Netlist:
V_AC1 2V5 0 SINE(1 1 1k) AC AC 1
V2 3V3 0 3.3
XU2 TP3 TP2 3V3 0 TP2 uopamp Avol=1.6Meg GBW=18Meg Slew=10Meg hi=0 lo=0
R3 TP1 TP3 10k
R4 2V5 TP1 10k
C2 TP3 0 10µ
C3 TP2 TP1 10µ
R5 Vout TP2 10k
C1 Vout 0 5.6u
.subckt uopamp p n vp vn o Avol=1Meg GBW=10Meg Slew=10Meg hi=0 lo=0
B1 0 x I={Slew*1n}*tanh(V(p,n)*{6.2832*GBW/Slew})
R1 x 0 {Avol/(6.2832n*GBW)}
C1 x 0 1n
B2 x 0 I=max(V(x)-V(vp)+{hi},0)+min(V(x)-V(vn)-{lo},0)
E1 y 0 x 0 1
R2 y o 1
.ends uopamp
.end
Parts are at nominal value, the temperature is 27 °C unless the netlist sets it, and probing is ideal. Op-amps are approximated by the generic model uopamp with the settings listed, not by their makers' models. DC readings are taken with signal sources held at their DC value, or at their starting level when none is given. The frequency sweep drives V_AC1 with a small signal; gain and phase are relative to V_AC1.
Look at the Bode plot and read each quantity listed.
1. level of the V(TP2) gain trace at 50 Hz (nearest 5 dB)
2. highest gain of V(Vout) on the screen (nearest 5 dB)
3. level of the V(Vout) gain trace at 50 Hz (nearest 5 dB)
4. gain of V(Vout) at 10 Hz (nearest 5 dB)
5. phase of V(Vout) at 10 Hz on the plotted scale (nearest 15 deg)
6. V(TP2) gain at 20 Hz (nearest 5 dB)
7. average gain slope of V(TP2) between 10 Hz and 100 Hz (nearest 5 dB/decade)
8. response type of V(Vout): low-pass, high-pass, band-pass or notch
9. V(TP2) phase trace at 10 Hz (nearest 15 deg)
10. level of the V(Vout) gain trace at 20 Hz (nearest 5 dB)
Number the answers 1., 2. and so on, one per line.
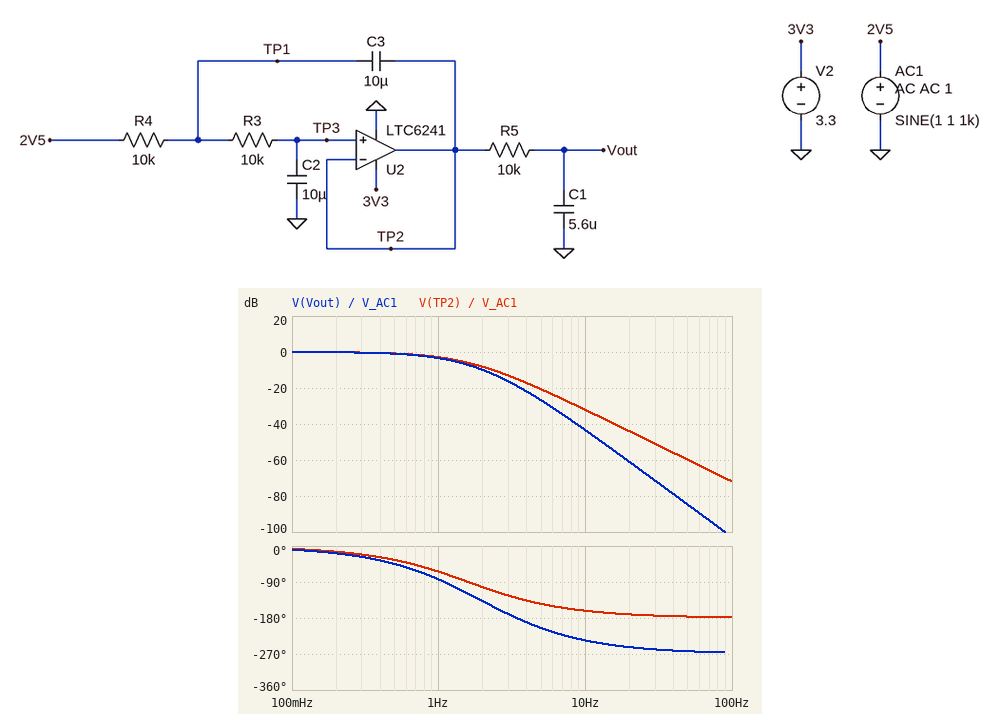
1. -60 dB
2. 0 dB
3. -85 dB
4. -45 dB
5. -240 deg
6. -45 dB
7. -40 dB/decade
8. low-pass
9. -165 deg
10. -60 dB
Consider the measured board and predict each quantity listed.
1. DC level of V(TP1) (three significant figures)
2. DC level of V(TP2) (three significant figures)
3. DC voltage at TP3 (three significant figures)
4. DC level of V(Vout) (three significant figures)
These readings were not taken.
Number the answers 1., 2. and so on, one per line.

1. 1.00 V
2. 1.00 V
3. 1.00 V
4. 1.00 V
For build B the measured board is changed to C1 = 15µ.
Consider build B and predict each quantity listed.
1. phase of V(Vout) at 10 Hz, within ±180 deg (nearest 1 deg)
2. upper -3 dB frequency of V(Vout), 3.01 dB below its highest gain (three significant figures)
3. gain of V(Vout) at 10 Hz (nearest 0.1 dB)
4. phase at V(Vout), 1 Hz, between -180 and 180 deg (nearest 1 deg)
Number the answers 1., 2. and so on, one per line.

1. 114 deg
2. 688 mHz
3. -51.7 dB
4. -108 deg
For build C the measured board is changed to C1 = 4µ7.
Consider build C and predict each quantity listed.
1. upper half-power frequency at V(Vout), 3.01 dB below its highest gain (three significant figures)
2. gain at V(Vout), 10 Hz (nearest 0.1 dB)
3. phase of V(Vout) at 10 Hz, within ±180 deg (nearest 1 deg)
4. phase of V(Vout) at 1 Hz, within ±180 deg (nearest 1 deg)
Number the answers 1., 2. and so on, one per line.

1. 956 mHz
2. -42.0 dB
3. 127 deg
4. -81 deg
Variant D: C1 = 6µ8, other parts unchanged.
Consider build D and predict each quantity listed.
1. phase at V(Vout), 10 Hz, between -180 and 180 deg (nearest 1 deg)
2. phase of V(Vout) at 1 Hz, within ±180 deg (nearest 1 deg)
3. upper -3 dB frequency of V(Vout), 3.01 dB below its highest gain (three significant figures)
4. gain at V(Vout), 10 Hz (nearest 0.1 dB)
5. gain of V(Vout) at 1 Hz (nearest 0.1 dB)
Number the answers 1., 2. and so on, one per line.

1. 121 deg
2. -87 deg
3. 900 mHz
4. -45.0 dB
5. -3.6 dB
